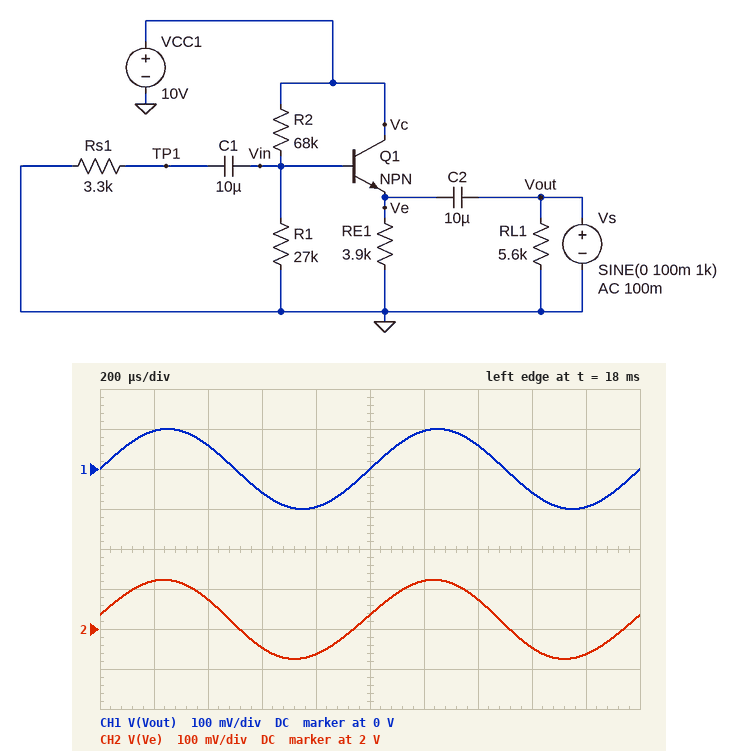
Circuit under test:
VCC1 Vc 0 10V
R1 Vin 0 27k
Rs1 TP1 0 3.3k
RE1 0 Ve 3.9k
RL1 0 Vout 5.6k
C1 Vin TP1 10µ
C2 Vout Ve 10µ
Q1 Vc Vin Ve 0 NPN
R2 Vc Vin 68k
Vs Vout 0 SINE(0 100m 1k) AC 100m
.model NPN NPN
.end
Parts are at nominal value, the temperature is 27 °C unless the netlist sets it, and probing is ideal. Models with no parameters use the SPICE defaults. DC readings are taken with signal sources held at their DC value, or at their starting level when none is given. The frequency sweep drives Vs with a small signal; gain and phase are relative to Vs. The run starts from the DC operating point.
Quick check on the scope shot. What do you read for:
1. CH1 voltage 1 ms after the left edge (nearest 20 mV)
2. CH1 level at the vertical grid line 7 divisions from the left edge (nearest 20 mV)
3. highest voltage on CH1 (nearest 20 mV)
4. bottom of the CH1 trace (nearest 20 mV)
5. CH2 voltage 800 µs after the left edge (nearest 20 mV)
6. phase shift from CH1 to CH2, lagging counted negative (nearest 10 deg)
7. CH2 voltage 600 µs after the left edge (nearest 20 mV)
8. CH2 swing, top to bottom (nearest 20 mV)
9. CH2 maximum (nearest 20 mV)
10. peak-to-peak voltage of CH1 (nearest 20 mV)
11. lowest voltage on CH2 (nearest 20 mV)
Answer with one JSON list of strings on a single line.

["0 V", "60 mV", "100 mV", "-100 mV", "1.94 V", "10 deg", "1.96 V", "200 mV", "2.12 V", "200 mV", "1.92 V"]
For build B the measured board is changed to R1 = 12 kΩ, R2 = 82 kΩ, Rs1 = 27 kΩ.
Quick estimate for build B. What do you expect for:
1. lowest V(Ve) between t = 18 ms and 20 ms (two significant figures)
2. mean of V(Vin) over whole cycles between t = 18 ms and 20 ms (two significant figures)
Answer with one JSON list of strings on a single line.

["480 mV", "1.3 V"]
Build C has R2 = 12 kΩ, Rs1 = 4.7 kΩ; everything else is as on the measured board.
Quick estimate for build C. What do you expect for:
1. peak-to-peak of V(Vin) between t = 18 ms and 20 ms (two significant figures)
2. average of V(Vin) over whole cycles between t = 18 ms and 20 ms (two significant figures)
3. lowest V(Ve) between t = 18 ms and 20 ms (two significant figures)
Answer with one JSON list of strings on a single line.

["100 mV", "6.8 V", "5.9 V"]
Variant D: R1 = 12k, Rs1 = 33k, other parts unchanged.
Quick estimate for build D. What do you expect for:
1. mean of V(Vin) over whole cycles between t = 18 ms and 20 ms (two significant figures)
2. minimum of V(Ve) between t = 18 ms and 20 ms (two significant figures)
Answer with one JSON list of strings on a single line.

["1.5 V", "680 mV"]
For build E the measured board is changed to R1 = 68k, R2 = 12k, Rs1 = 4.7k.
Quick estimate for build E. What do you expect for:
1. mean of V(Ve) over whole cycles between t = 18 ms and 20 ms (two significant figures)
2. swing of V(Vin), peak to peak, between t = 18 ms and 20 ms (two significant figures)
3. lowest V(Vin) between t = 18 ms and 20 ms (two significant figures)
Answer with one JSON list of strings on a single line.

["7.5 V", "120 mV", "8.2 V"]
